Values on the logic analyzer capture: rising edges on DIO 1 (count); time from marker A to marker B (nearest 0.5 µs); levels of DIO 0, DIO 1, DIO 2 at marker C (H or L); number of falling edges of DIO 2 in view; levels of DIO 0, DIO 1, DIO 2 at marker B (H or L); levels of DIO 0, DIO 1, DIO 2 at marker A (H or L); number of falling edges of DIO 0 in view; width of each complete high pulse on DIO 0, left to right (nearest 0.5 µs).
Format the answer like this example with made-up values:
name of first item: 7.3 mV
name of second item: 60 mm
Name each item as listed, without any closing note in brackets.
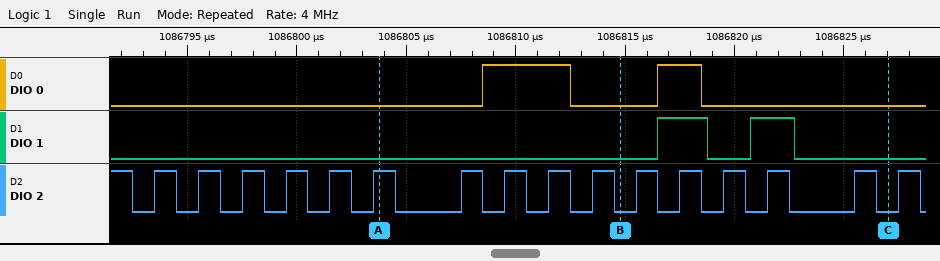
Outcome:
rising edges on DIO 1: 2
time from marker A to marker B: 11 µs
levels of DIO 0, DIO 1, DIO 2 at marker C: DIO 0=L, DIO 1=L, DIO 2=L
number of falling edges of DIO 2 in view: 17
levels of DIO 0, DIO 1, DIO 2 at marker B: DIO 0=L, DIO 1=L, DIO 2=L
levels of DIO 0, DIO 1, DIO 2 at marker A: DIO 0=L, DIO 1=L, DIO 2=H
number of falling edges of DIO 0 in view: 2
width of each complete high pulse on DIO 0, left to right: 4 µs, 2 µs
